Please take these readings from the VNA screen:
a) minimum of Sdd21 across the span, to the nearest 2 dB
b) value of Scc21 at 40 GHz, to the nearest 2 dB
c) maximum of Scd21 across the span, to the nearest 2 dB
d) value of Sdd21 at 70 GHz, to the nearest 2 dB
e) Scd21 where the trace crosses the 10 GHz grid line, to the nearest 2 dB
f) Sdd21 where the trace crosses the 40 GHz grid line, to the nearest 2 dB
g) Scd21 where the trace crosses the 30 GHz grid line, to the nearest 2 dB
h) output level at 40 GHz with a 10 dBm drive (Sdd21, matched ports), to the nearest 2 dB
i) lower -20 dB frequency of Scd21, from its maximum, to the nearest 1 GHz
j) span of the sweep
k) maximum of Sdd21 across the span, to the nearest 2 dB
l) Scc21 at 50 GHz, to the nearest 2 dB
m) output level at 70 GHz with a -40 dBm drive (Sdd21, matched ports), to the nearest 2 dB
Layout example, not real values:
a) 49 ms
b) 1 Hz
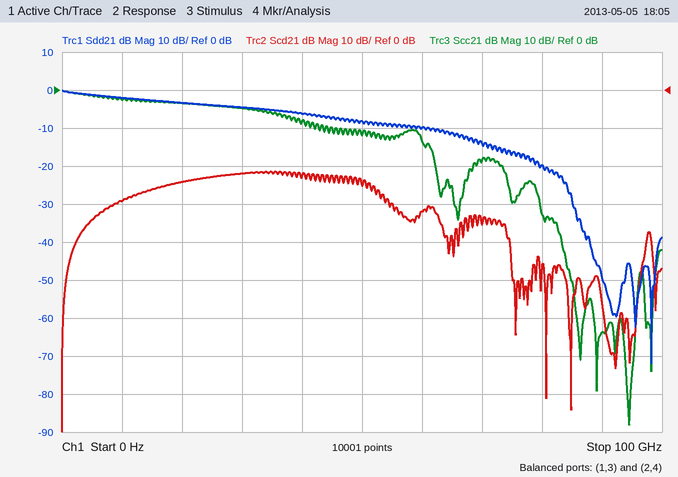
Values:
a) -72 dB
b) -8 dB
c) -22 dB
d) -14 dB
e) -30 dB
f) -6 dB
g) -22 dB
h) 4 dBm
i) 2 GHz
j) 100 GHz
k) 0 dB
l) -12 dB
m) -54 dBm
